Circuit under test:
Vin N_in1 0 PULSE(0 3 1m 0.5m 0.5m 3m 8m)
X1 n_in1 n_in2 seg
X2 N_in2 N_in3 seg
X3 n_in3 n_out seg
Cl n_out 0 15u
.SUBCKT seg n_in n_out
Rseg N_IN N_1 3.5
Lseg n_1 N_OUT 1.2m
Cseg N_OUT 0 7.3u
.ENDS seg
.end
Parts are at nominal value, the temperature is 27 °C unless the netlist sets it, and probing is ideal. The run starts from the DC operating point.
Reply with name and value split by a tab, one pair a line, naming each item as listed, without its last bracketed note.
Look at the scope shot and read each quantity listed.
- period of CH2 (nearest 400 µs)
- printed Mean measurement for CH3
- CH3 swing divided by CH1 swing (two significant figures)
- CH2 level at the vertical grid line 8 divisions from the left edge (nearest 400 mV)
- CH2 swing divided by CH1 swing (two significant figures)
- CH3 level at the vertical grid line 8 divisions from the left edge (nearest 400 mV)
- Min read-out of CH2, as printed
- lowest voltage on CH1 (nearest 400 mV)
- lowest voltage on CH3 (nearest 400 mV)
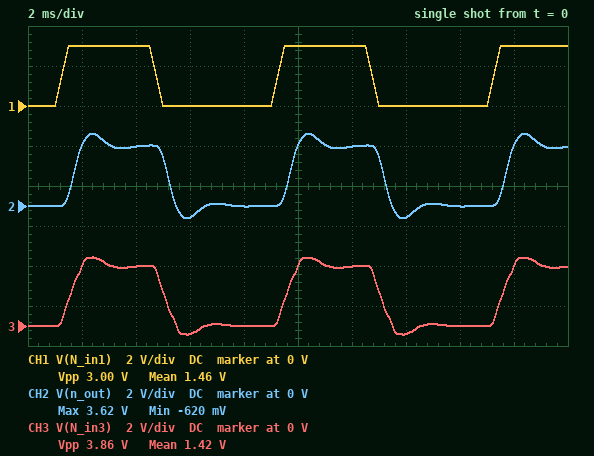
period of CH2	8.0 ms
printed Mean measurement for CH3	1.42 V
CH3 swing divided by CH1 swing	1.3
CH2 level at the vertical grid line 8 divisions from the left edge	0 V
CH2 swing divided by CH1 swing	1.4
CH3 level at the vertical grid line 8 divisions from the left edge	0 V
Min read-out of CH2, as printed	-620 mV
lowest voltage on CH1	0 V
lowest voltage on CH3	-400 mV
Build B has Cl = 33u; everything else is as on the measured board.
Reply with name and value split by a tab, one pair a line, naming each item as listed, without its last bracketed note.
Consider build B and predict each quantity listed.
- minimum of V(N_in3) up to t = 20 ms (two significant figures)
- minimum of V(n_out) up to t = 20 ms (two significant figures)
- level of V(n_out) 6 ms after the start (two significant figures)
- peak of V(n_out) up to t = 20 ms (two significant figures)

minimum of V(N_in3) up to t = 20 ms	-250 mV
minimum of V(n_out) up to t = 20 ms	-310 mV
level of V(n_out) 6 ms after the start	-170 mV
peak of V(n_out) up to t = 20 ms	3.3 V
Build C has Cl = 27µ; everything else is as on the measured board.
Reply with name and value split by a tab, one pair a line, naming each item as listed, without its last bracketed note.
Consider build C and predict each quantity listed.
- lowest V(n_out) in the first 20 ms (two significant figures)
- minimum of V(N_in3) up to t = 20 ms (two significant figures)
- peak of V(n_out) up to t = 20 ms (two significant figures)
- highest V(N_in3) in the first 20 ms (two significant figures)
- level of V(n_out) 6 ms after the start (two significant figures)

lowest V(n_out) in the first 20 ms	-390 mV
minimum of V(N_in3) up to t = 20 ms	-310 mV
peak of V(n_out) up to t = 20 ms	3.4 V
highest V(N_in3) in the first 20 ms	3.3 V
level of V(n_out) 6 ms after the start	-350 mV
